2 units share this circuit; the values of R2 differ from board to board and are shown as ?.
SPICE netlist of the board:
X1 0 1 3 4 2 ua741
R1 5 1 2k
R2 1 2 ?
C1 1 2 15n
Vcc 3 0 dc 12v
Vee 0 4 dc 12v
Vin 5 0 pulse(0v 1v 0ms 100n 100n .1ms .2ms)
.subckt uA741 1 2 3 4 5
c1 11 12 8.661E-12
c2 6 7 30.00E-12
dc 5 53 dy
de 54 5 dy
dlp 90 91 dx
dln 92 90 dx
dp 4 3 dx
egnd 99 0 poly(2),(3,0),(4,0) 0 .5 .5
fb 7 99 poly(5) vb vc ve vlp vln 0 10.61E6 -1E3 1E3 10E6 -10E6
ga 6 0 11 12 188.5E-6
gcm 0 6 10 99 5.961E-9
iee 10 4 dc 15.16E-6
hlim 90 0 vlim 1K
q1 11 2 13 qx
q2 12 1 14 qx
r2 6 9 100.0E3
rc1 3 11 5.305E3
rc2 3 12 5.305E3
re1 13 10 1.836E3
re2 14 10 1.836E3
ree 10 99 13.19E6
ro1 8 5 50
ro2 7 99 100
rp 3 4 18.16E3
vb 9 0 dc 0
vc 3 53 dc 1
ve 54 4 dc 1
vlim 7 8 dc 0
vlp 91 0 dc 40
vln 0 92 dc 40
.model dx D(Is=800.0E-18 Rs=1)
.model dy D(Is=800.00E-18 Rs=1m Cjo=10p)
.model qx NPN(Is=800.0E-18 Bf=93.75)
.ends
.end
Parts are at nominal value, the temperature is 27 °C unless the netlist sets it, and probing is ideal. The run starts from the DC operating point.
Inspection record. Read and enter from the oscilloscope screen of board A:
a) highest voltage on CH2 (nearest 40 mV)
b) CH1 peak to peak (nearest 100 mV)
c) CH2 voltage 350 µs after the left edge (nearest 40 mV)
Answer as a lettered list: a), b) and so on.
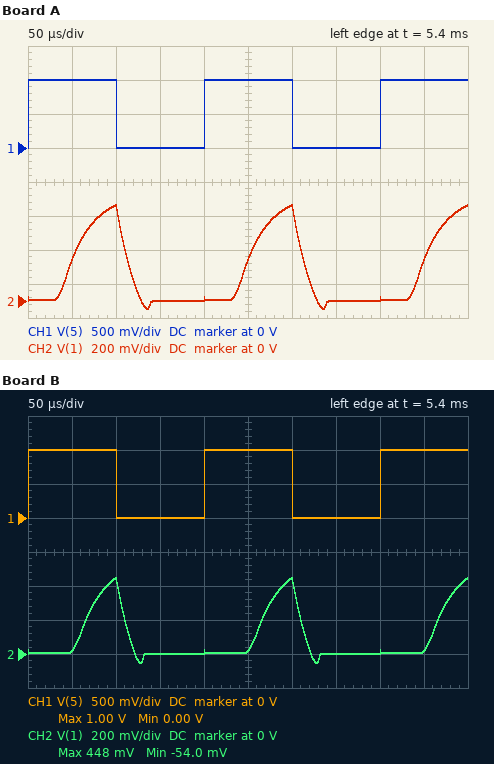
a) 560 mV
b) 1.0 V
c) 0 V
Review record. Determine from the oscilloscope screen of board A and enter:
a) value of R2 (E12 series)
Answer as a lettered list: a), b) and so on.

a) 68 kΩ
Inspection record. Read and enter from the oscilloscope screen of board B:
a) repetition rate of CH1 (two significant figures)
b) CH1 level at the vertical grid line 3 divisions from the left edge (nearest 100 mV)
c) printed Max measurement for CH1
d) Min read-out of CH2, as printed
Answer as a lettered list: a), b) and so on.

a) 5.0 kHz
b) 0 V
c) 1.00 V
d) -54.0 mV
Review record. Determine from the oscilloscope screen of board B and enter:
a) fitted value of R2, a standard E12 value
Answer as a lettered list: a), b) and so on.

a) 56 kΩ
